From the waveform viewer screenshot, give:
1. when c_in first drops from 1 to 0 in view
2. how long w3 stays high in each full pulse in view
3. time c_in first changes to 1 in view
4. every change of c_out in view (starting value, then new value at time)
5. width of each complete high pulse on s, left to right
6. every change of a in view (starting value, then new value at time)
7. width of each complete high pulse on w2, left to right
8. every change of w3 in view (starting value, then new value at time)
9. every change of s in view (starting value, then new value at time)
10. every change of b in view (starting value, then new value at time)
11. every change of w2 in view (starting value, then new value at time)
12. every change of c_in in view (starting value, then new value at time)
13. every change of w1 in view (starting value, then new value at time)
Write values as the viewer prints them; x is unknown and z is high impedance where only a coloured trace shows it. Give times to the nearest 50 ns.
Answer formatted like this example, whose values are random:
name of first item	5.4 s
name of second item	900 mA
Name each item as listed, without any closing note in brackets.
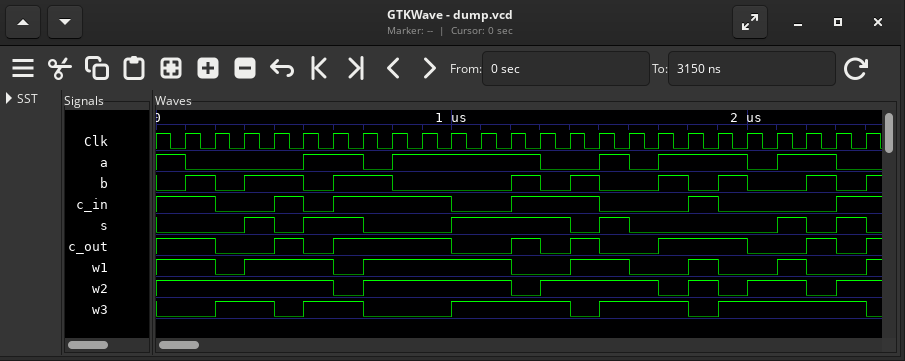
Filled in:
when c_in first drops from 1 to 0 in view	200 ns
how long w3 stays high in each full pulse in view	200 ns, 200 ns, 400 ns, 300 ns, 500 ns
time c_in first changes to 1 in view	400 ns
every change of c_out in view	1, 0 at 200 ns, 1 at 400 ns, 0 at 500 ns, 1 at 600 ns, 0 at 1000 ns, 1 at 1200 ns, 0 at 1300 ns, 1 at 1400 ns, 0 at 1500 ns, 1 at 1700 ns, 0 at 2000 ns, 1 at 2200 ns, 0 at 2300 ns, 1 at 2400 ns
width of each complete high pulse on s, left to right	100 ns, 200 ns, 400 ns, 100 ns, 100 ns, 100 ns
every change of a in view	1, 0 at 100 ns, 1 at 500 ns, 0 at 700 ns, 1 at 800 ns, 0 at 1300 ns, 1 at 1500 ns, 0 at 1600 ns, 1 at 1700 ns, 0 at 2000 ns, 1 at 2100 ns, 0 at 2300 ns
width of each complete high pulse on w2, left to right	500 ns, 400 ns, 100 ns, 200 ns
every change of w3 in view	0, 1 at 200 ns, 0 at 400 ns, 1 at 500 ns, 0 at 700 ns, 1 at 1000 ns, 0 at 1400 ns, 1 at 1500 ns, 0 at 1800 ns, 1 at 1900 ns, 0 at 2400 ns
every change of s in view	0, 1 at 300 ns, 0 at 400 ns, 1 at 500 ns, 0 at 700 ns, 1 at 1000 ns, 0 at 1400 ns, 1 at 1500 ns, 0 at 1600 ns, 1 at 2100 ns, 0 at 2200 ns, 1 at 2300 ns, 0 at 2400 ns
every change of b in view	0, 1 at 100 ns, 0 at 200 ns, 1 at 300 ns, 0 at 500 ns, 1 at 600 ns, 0 at 800 ns, 1 at 1200 ns, 0 at 1300 ns, 1 at 1400 ns, 0 at 1500 ns, 1 at 1700 ns, 0 at 1800 ns, 1 at 1900 ns, 0 at 2000 ns, 1 at 2200 ns, 0 at 2300 ns, 1 at 2400 ns
every change of w2 in view	1, 0 at 600 ns, 1 at 700 ns, 0 at 1200 ns, 1 at 1300 ns, 0 at 1700 ns, 1 at 1800 ns, 0 at 1900 ns, 1 at 2000 ns, 0 at 2200 ns, 1 at 2300 ns
every change of c_in in view	1, 0 at 200 ns, 1 at 400 ns, 0 at 500 ns, 1 at 600 ns, 0 at 1000 ns, 1 at 1200 ns, 0 at 1500 ns, 1 at 1800 ns, 0 at 1900 ns, 1 at 2300 ns
every change of w1 in view	1, 0 at 200 ns, 1 at 300 ns, 0 at 600 ns, 1 at 700 ns, 0 at 1200 ns, 1 at 1400 ns, 0 at 1600 ns, 1 at 1800 ns, 0 at 1900 ns, 1 at 2100 ns, 0 at 2200 ns, 1 at 2400 ns
